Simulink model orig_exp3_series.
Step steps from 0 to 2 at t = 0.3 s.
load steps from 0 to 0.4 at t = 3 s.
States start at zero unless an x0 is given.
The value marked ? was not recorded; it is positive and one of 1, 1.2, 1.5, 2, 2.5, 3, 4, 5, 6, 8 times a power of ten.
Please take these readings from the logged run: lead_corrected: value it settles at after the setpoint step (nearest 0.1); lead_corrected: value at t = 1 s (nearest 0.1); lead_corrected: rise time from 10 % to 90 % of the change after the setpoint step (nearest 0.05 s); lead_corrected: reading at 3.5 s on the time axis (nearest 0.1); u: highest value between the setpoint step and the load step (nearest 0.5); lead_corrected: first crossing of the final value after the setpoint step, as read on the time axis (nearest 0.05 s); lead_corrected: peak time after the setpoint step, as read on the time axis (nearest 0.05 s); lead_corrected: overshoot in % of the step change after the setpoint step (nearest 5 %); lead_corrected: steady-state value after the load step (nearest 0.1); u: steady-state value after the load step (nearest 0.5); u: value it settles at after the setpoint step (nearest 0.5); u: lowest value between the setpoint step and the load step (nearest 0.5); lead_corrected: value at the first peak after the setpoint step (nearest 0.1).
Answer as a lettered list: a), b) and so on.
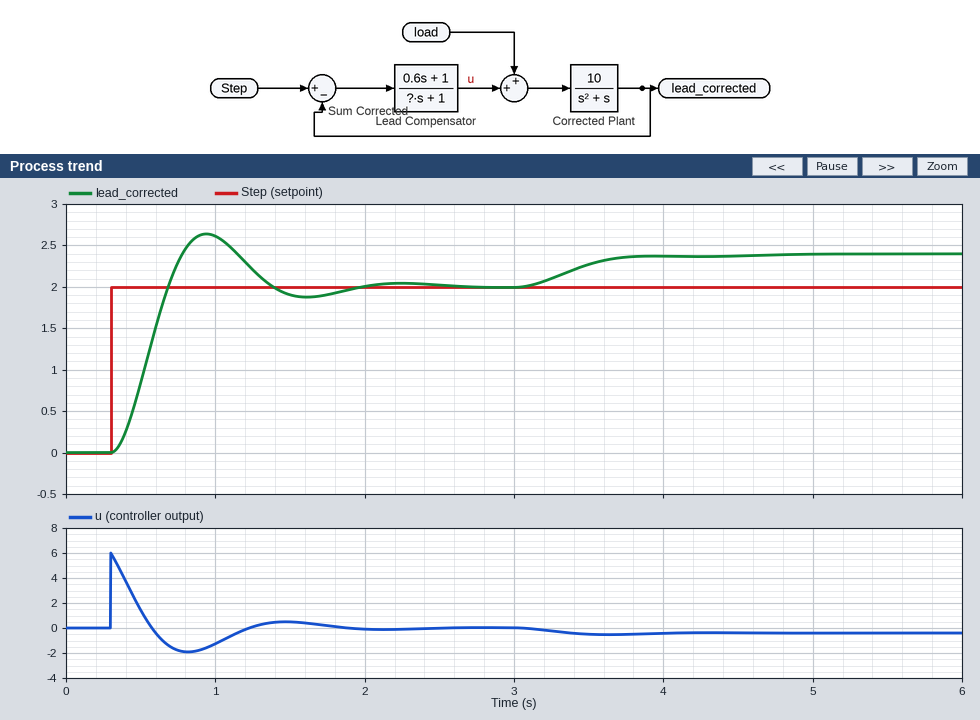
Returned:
a) 2.0
b) 2.6
c) 0.25 s
d) 2.3
e) 6.0
f) 0.70 s
g) 0.95 s
h) 30 %
i) 2.4
j) -0.5
k) 0.0
l) -2.0
m) 2.6
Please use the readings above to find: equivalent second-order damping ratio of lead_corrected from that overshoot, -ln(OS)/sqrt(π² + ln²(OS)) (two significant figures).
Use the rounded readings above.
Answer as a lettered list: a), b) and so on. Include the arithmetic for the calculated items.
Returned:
a) ln(0.3) = -1.204; 1.204 / sqrt(9.870 + 1.450) = 0.36
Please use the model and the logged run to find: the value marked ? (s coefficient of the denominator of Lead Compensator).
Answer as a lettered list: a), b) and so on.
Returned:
a) 0.2
